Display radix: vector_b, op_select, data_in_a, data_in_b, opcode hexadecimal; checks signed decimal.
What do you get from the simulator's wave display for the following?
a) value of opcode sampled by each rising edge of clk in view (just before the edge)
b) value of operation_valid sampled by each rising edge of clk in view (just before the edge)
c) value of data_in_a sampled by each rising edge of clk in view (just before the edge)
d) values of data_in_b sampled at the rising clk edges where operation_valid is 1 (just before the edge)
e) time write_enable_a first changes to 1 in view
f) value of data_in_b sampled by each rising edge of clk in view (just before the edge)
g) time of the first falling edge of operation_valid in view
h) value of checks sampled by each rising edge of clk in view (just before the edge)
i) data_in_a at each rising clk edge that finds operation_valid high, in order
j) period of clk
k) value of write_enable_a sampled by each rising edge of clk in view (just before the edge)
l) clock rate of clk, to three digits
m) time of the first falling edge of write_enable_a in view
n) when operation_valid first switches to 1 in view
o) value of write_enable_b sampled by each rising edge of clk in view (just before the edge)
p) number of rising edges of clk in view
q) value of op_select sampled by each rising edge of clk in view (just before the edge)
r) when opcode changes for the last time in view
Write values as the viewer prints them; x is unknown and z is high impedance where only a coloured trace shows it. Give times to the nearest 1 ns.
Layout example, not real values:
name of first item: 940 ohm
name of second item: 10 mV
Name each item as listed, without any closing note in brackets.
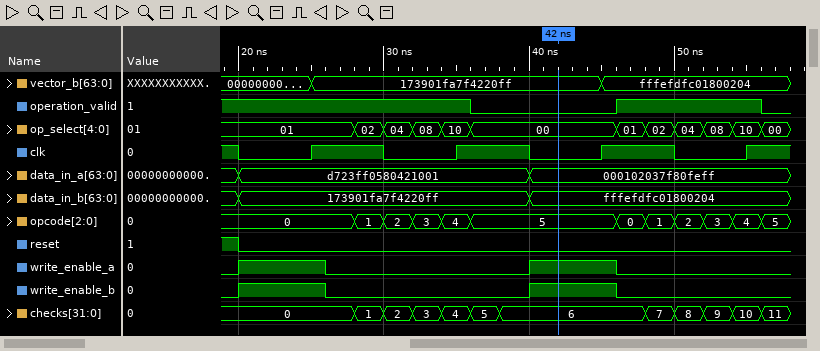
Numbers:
value of opcode sampled by each rising edge of clk in view: 0, 4, 5, 4
value of operation_valid sampled by each rising edge of clk in view: 1 1 0 1
value of data_in_a sampled by each rising edge of clk in view: d723ff0580421001, d723ff0580421001, 000102037f80feff, 000102037f80feff
values of data_in_b sampled at the rising clk edges where operation_valid is 1: 173901fa7f4220ff, 173901fa7f4220ff, fffefdfc01800204
time write_enable_a first changes to 1 in view: 20 ns
value of data_in_b sampled by each rising edge of clk in view: 173901fa7f4220ff, 173901fa7f4220ff, fffefdfc01800204, fffefdfc01800204
time of the first falling edge of operation_valid in view: 36 ns
value of checks sampled by each rising edge of clk in view: 0, 4, 6, 10
data_in_a at each rising clk edge that finds operation_valid high, in order: d723ff0580421001, d723ff0580421001, 000102037f80feff
period of clk: 10 ns
value of write_enable_a sampled by each rising edge of clk in view: 1 0 1 0
clock rate of clk, to three digits: 100 MHz
time of the first falling edge of write_enable_a in view: 26 ns
when operation_valid first switches to 1 in view: 46 ns
value of write_enable_b sampled by each rising edge of clk in view: 1 0 1 0
number of rising edges of clk in view: 4
value of op_select sampled by each rising edge of clk in view: 01, 10, 00, 10
when opcode changes for the last time in view: 56 ns
